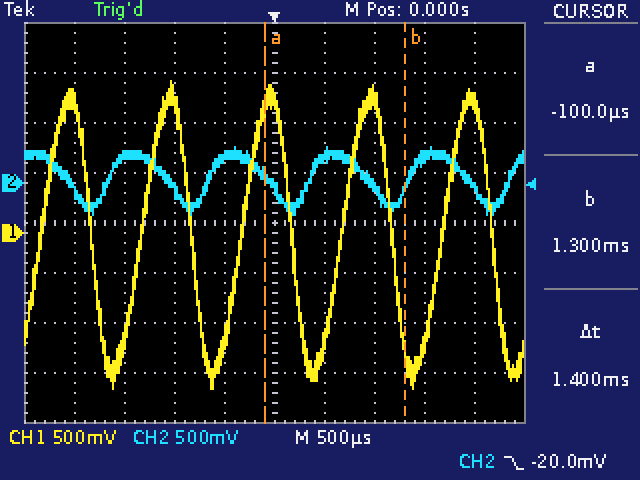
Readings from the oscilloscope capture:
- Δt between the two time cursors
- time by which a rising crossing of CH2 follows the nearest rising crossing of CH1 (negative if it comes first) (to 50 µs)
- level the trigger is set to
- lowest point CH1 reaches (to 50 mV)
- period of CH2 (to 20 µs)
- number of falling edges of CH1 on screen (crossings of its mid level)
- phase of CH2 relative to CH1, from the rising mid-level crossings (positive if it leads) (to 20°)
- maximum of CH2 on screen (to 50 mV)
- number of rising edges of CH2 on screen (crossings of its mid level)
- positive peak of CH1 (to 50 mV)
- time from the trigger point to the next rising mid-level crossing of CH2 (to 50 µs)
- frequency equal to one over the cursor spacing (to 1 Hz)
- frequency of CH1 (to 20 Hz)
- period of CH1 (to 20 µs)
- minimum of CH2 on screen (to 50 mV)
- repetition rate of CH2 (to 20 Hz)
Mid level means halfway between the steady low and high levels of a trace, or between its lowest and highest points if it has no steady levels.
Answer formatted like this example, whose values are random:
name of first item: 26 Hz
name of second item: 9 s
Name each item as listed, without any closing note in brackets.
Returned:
Δt between the two time cursors: 1.4 ms
time by which a rising crossing of CH2 follows the nearest rising crossing of CH1 (negative if it comes first): -350 µs
level the trigger is set to: -20.0 mV
lowest point CH1 reaches: -1.55 V
period of CH2: 1.00 ms
number of falling edges of CH1 on screen: 5
phase of CH2 relative to CH1, from the rising mid-level crossings (positive if it leads): +120°
maximum of CH2 on screen: 350 mV
number of rising edges of CH2 on screen: 5
positive peak of CH1: 1.50 V
time from the trigger point to the next rising mid-level crossing of CH2: 350 µs
frequency equal to one over the cursor spacing: 714 Hz
frequency of CH1: 1.00 kHz
period of CH1: 1.00 ms
minimum of CH2 on screen: -300 mV
repetition rate of CH2: 1.00 kHz
